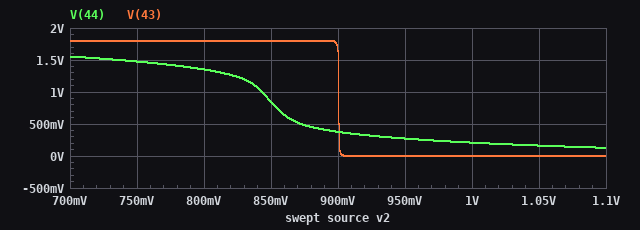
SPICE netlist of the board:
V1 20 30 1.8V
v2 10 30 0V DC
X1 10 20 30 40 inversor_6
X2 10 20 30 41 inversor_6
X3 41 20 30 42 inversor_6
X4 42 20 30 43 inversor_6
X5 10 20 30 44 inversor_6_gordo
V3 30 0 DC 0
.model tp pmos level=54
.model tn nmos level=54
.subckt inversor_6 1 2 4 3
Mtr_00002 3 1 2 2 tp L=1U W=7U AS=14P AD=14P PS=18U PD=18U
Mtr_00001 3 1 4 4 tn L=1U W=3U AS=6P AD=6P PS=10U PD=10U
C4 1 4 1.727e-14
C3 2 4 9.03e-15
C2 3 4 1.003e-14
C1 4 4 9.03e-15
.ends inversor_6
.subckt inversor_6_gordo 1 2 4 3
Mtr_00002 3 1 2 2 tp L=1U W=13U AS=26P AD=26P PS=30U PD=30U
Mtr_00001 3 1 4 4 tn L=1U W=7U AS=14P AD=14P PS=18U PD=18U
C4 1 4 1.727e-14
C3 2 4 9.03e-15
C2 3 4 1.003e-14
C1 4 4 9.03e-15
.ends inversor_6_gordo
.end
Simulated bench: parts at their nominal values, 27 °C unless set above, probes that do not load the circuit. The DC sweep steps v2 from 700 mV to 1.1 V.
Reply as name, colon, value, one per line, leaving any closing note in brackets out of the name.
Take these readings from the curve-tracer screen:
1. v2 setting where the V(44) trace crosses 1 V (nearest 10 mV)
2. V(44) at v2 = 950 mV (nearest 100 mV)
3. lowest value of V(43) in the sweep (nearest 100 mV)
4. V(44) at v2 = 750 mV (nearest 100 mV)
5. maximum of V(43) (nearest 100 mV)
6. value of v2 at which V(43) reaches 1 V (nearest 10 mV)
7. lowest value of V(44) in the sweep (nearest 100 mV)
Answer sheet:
v2 setting where the V(44) trace crosses 1 V: 840 mV
V(44) at v2 = 950 mV: 300 mV
lowest value of V(43) in the sweep: 0 V
V(44) at v2 = 750 mV: 1.5 V
maximum of V(43): 1.8 V
value of v2 at which V(43) reaches 1 V: 900 mV
lowest value of V(44) in the sweep: 100 mV
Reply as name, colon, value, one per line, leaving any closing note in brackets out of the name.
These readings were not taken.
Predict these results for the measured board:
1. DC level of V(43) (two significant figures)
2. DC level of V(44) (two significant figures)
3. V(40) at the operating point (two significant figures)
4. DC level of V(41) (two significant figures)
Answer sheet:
DC level of V(43): 1.8 V
DC level of V(44): 1.8 V
V(40) at the operating point: 1.8 V
DC level of V(41): 1.8 V
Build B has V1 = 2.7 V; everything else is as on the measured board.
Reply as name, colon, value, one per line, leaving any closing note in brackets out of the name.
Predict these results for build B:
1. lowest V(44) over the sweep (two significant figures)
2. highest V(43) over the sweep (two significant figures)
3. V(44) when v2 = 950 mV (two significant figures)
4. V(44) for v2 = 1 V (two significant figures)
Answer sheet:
lowest V(44) over the sweep: 2.2 V
highest V(43) over the sweep: 2.7 V
V(44) when v2 = 950 mV: 2.4 V
V(44) for v2 = 1 V: 2.3 V
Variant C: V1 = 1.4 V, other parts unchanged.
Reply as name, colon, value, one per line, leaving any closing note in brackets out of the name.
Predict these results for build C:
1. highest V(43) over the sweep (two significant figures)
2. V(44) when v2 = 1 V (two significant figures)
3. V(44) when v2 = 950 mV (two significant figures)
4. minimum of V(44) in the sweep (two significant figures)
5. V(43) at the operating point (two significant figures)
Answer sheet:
highest V(43) over the sweep: 24 mV
V(44) when v2 = 1 V: 25 mV
V(44) when v2 = 950 mV: 40 mV
minimum of V(44) in the sweep: 6.2 mV
V(43) at the operating point: 1.4 V
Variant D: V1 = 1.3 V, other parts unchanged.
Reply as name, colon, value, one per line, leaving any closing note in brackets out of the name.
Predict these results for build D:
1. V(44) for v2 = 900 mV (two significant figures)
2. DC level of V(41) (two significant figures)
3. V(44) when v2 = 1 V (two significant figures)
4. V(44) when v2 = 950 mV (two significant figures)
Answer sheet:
V(44) for v2 = 900 mV: 28 mV
DC level of V(41): 1.3 V
V(44) when v2 = 1 V: 6.8 mV
V(44) when v2 = 950 mV: 15 mV
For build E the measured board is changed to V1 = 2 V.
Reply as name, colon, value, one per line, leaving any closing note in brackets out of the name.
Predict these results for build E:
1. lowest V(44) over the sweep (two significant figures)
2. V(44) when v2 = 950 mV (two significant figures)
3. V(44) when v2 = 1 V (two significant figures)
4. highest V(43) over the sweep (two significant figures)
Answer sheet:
lowest V(44) over the sweep: 250 mV
V(44) when v2 = 950 mV: 810 mV
V(44) when v2 = 1 V: 430 mV
highest V(43) over the sweep: 2.0 V
